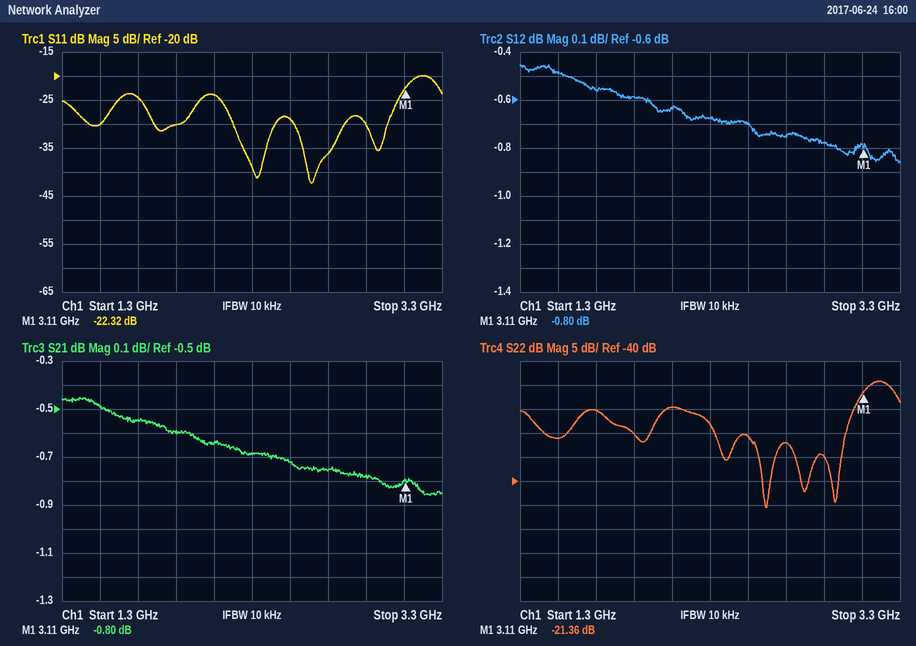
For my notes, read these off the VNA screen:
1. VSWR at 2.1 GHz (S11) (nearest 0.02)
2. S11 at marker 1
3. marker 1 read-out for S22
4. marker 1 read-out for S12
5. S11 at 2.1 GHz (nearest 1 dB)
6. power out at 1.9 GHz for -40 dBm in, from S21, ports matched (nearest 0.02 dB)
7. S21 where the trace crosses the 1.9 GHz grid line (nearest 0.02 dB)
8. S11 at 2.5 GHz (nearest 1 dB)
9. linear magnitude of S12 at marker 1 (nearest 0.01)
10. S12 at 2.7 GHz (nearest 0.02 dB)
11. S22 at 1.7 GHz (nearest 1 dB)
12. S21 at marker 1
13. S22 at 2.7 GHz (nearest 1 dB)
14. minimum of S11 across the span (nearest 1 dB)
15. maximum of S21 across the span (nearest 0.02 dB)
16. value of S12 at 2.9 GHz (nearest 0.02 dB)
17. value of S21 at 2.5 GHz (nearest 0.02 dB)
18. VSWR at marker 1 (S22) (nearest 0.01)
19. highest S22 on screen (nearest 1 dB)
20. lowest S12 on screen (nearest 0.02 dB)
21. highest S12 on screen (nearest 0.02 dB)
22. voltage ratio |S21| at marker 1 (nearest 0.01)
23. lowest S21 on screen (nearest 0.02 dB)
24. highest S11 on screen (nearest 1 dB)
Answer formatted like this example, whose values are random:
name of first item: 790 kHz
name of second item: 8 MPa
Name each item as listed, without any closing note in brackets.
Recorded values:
VSWR at 2.1 GHz (S11): 1.14
S11 at marker 1: -22.32 dB
marker 1 read-out for S22: -21.36 dB
marker 1 read-out for S12: -0.80 dB
S11 at 2.1 GHz: -24 dB
power out at 1.9 GHz for -40 dBm in, from S21, ports matched: -40.60 dBm
S21 where the trace crosses the 1.9 GHz grid line: -0.60 dB
S11 at 2.5 GHz: -29 dB
linear magnitude of S12 at marker 1: 0.91
S12 at 2.7 GHz: -0.74 dB
S22 at 1.7 GHz: -25 dB
S21 at marker 1: -0.80 dB
S22 at 2.7 GHz: -32 dB
minimum of S11 across the span: -42 dB
maximum of S21 across the span: -0.46 dB
value of S12 at 2.9 GHz: -0.78 dB
value of S21 at 2.5 GHz: -0.72 dB
VSWR at marker 1 (S22): 1.19
highest S22 on screen: -19 dB
lowest S12 on screen: -0.86 dB
highest S12 on screen: -0.46 dB
voltage ratio |S21| at marker 1: 0.91
lowest S21 on screen: -0.86 dB
highest S11 on screen: -20 dB
